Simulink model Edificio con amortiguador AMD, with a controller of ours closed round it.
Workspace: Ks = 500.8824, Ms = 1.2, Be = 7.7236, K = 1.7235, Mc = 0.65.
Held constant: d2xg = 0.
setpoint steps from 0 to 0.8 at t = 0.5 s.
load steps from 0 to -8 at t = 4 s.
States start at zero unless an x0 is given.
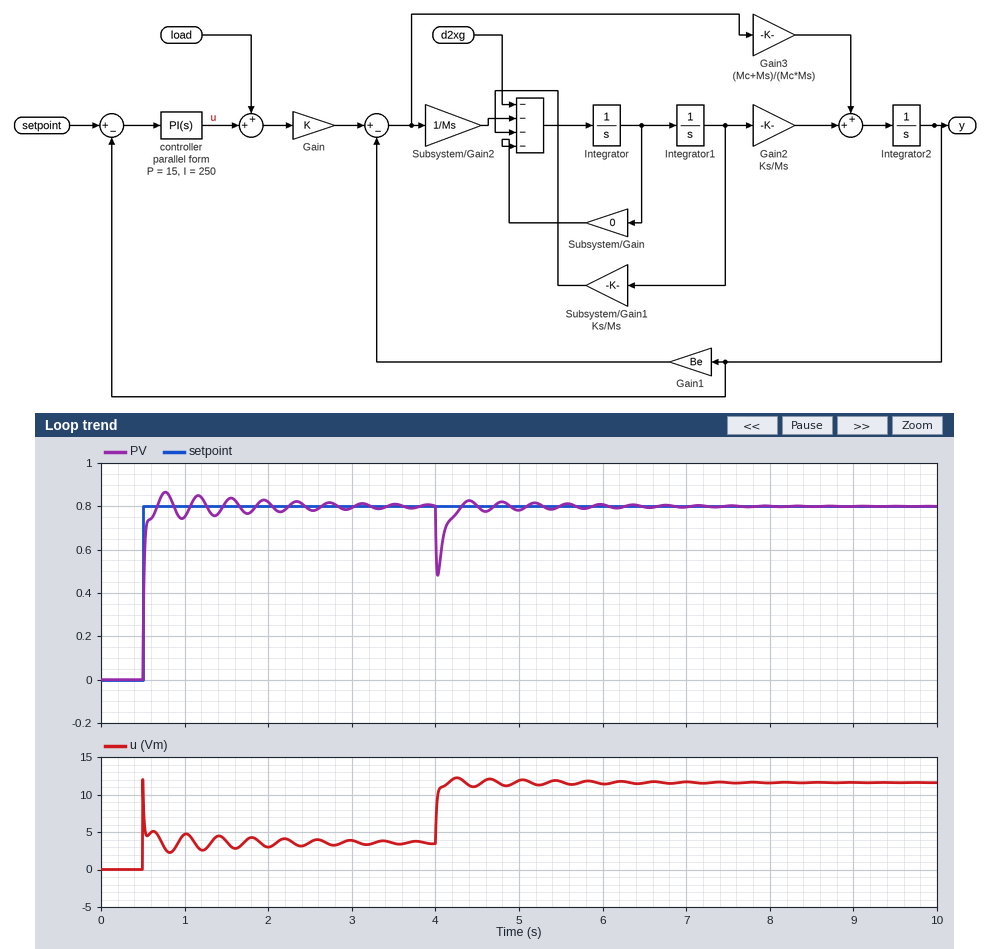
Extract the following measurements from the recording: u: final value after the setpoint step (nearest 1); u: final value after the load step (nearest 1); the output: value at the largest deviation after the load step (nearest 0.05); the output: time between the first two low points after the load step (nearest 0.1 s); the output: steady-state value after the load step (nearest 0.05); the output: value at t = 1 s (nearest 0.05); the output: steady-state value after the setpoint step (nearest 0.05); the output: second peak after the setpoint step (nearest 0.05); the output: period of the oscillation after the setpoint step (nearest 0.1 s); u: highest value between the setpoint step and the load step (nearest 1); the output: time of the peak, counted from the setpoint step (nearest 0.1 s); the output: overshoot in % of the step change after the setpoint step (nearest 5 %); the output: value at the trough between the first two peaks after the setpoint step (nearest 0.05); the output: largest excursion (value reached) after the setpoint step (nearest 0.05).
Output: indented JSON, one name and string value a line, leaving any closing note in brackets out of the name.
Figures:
{
  "u: final value after the setpoint step": "4",
  "u: final value after the load step": "12",
  "the output: value at the largest deviation after the load step": "0.50",
  "the output: time between the first two low points after the load step": "0.6 s",
  "the output: steady-state value after the load step": "0.80",
  "the output: value at t = 1 s": "0.75",
  "the output: steady-state value after the setpoint step": "0.80",
  "the output: second peak after the setpoint step": "0.85",
  "the output: period of the oscillation after the setpoint step": "0.4 s",
  "u: highest value between the setpoint step and the load step": "12",
  "the output: time of the peak, counted from the setpoint step": "0.3 s",
  "the output: overshoot in % of the step change after the setpoint step": "10 %",
  "the output: value at the trough between the first two peaks after the setpoint step": "0.75",
  "the output: largest excursion (value reached) after the setpoint step": "0.85"
}
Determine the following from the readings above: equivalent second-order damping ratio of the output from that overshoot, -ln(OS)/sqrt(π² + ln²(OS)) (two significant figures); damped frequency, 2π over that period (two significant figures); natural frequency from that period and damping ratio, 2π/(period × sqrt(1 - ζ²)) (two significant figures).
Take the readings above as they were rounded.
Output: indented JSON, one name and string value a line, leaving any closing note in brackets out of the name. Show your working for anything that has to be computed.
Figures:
{
  "equivalent second-order damping ratio of the output from that overshoot, -ln(OS)/sqrt(π² + ln²(OS))": "ln(0.1) = -2.303; 2.303 / sqrt(9.870 + 5.302) = 0.59",
  "damped frequency, 2π over that period": "2π / 0.4 = 16 rad/s",
  "natural frequency from that period and damping ratio, 2π/(period × sqrt(1 - ζ²))": "2π / (0.4 × sqrt(1 - 0.59²)) = 19 rad/s"
}
